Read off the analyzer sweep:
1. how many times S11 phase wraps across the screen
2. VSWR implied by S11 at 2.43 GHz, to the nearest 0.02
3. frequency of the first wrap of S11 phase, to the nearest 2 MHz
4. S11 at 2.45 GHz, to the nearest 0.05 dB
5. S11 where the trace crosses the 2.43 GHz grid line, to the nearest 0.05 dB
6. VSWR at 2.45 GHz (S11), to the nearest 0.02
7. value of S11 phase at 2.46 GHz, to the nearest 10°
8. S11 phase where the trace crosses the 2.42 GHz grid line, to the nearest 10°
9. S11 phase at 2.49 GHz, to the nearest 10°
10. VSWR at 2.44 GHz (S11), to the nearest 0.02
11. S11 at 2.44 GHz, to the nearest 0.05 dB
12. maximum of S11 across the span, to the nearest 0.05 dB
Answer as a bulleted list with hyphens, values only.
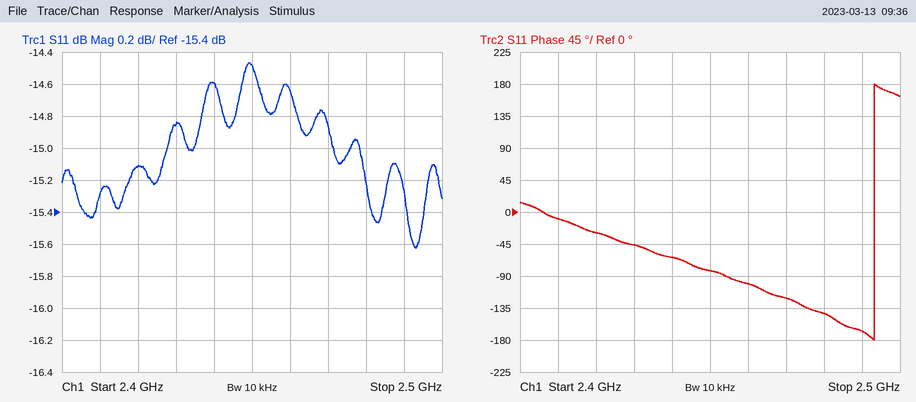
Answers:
- 1
- 1.44
- 2.494 GHz
- -14.50 dB
- -14.85 dB
- 1.46
- -100°
- -30°
- -170°
- 1.46
- -14.60 dB
- -14.45 dB
